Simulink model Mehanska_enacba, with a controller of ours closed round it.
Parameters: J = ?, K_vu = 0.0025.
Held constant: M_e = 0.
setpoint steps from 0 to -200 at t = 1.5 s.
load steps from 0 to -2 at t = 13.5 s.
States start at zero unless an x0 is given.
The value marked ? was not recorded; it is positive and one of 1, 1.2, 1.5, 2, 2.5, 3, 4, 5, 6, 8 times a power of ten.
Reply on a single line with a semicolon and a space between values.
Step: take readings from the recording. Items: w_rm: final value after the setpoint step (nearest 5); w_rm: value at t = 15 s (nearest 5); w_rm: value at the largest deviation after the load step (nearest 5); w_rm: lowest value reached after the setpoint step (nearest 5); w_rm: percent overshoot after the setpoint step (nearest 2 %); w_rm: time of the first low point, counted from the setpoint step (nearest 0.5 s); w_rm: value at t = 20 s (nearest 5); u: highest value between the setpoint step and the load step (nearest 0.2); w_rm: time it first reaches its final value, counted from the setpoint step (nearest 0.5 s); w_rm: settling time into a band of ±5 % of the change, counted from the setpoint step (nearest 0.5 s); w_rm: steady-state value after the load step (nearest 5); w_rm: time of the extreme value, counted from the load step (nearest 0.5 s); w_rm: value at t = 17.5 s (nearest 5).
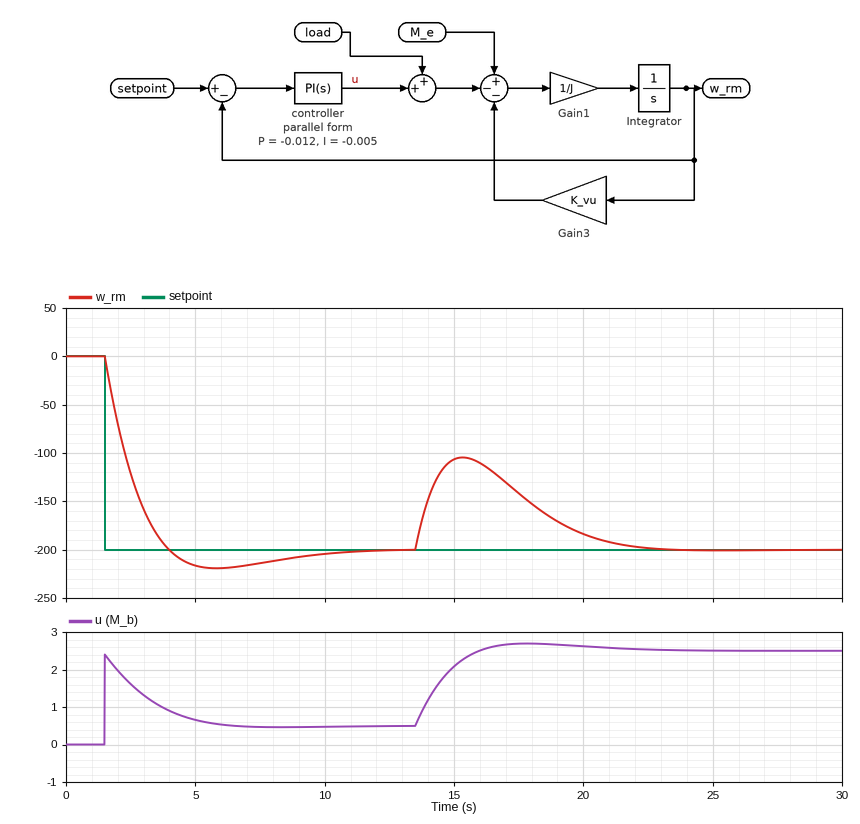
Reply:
-200; -105; -105; -220; 10 %; 4.5 s; -185; 2.4; 2.5 s; 7.0 s; -200; 2.0 s; -140
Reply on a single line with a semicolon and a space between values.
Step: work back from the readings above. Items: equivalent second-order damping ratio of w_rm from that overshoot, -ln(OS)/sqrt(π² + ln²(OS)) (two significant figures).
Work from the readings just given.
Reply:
0.59
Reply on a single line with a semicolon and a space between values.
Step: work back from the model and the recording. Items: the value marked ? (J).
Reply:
0.015
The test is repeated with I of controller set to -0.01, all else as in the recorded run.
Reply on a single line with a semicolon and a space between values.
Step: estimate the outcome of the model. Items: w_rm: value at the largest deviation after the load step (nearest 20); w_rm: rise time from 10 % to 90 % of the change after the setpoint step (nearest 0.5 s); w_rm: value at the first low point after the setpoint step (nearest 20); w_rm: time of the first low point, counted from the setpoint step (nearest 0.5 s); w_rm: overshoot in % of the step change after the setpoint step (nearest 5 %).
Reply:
-120; 1.5 s; -240; 3.0 s; 20 %
